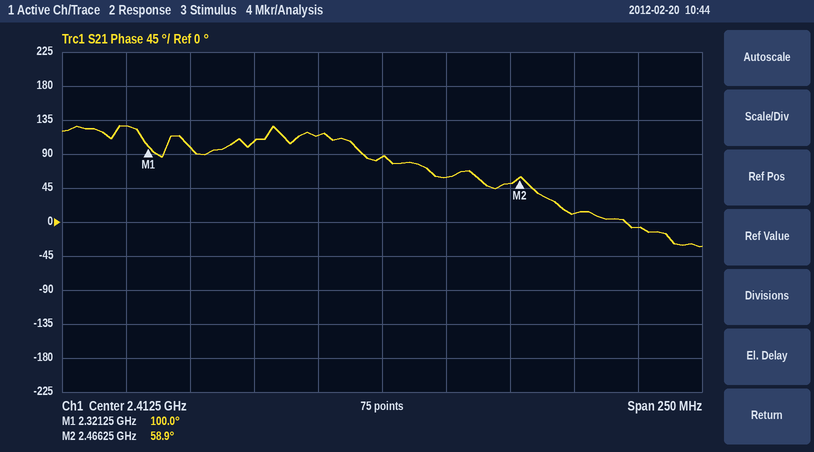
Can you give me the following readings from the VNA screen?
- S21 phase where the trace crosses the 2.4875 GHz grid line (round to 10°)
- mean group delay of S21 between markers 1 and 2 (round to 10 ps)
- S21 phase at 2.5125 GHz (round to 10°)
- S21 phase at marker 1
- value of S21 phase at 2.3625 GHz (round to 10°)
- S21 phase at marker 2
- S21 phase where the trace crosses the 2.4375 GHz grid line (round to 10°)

10°
790 ps
-10°
100.0°
110°
58.9°
60°
